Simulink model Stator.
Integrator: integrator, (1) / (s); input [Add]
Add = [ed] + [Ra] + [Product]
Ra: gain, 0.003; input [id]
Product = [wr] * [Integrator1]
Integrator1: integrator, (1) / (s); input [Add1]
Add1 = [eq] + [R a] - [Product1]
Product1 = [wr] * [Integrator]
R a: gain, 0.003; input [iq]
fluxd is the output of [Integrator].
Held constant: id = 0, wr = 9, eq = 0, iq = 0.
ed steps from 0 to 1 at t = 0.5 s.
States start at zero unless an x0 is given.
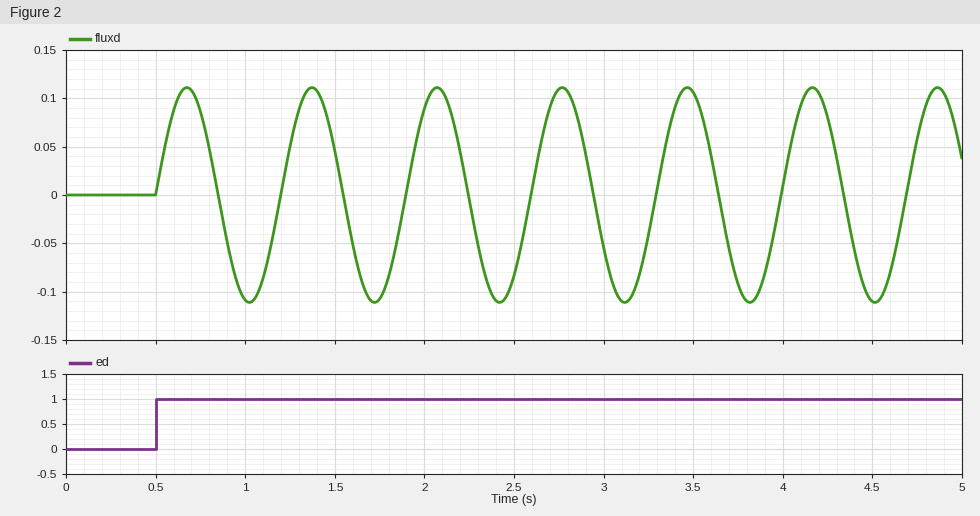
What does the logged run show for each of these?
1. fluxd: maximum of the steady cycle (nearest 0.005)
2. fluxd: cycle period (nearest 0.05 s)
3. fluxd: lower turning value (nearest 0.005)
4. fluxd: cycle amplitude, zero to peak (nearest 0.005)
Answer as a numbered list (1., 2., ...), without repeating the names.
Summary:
1. 0.110
2. 0.70 s
3. -0.110
4. 0.110
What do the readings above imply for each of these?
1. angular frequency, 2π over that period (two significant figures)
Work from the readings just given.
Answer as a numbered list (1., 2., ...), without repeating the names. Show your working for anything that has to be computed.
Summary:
1. 2π / 0.7 = 9.0 rad/s
